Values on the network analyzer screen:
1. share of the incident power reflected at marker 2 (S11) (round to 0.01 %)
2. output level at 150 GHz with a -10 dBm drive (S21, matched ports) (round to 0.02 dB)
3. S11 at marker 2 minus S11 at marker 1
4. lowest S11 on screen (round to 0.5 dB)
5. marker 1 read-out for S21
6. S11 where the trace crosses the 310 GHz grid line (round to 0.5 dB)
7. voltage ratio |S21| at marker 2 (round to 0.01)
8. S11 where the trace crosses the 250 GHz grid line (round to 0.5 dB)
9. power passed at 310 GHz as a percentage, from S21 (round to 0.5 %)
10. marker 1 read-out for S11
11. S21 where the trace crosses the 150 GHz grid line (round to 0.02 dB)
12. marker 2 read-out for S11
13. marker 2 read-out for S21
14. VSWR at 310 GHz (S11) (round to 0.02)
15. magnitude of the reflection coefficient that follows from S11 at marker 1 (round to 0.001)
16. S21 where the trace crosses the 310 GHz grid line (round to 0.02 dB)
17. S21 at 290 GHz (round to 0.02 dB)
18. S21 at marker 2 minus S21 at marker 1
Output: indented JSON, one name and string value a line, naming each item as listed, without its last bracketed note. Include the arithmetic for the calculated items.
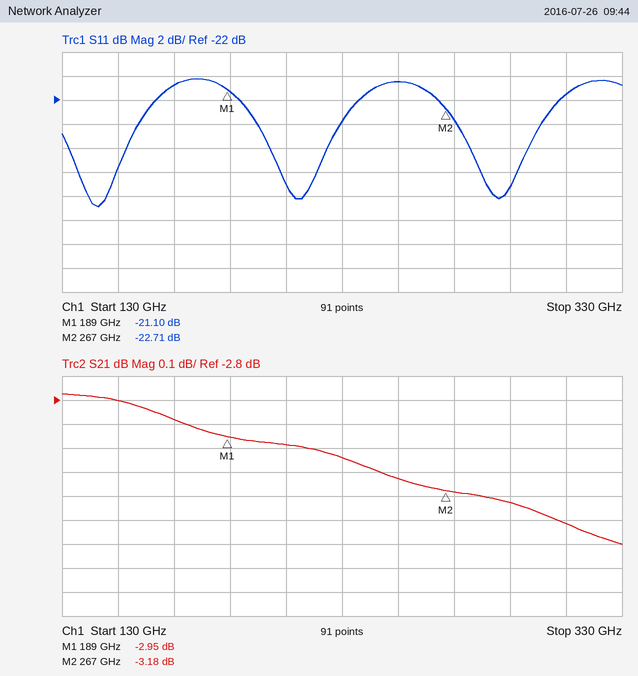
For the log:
{
  "share of the incident power reflected at marker 2 (S11)": "10^(-22.71/10) ≈ 0.54 %",
  "output level at 150 GHz with a -10 dBm drive (S21, matched ports)": "-10 dBm + (-2.80 dB) = -12.80 dBm",
  "S11 at marker 2 minus S11 at marker 1": "-22.71 − (-21.1) = -1.61 dB",
  "lowest S11 on screen": "-31.0 dB",
  "marker 1 read-out for S21": "-2.95 dB",
  "S11 where the trace crosses the 310 GHz grid line": "-21.5 dB",
  "voltage ratio |S21| at marker 2": "10^(-3.18/20) ≈ 0.69",
  "S11 where the trace crosses the 250 GHz grid line": "-20.5 dB",
  "power passed at 310 GHz as a percentage, from S21": "10^(-3.32/10) ≈ 46.6 %, so 46.5 % to the nearest 0.5 %",
  "marker 1 read-out for S11": "-21.10 dB",
  "S21 where the trace crosses the 150 GHz grid line": "-2.80 dB",
  "marker 2 read-out for S11": "-22.71 dB",
  "marker 2 read-out for S21": "-3.18 dB",
  "VSWR at 310 GHz (S11)": "|Γ| = 10^(-21.5/20) = 0.0841; VSWR = (1 + 0.0841)/(1 − 0.0841) ≈ 1.18",
  "magnitude of the reflection coefficient that follows from S11 at marker 1": "10^(-21.1/20) ≈ 0.088",
  "S21 where the trace crosses the 310 GHz grid line": "-3.32 dB",
  "S21 at 290 GHz": "-3.22 dB",
  "S21 at marker 2 minus S21 at marker 1": "-3.18 − (-2.95) = -0.23 dB"
}
